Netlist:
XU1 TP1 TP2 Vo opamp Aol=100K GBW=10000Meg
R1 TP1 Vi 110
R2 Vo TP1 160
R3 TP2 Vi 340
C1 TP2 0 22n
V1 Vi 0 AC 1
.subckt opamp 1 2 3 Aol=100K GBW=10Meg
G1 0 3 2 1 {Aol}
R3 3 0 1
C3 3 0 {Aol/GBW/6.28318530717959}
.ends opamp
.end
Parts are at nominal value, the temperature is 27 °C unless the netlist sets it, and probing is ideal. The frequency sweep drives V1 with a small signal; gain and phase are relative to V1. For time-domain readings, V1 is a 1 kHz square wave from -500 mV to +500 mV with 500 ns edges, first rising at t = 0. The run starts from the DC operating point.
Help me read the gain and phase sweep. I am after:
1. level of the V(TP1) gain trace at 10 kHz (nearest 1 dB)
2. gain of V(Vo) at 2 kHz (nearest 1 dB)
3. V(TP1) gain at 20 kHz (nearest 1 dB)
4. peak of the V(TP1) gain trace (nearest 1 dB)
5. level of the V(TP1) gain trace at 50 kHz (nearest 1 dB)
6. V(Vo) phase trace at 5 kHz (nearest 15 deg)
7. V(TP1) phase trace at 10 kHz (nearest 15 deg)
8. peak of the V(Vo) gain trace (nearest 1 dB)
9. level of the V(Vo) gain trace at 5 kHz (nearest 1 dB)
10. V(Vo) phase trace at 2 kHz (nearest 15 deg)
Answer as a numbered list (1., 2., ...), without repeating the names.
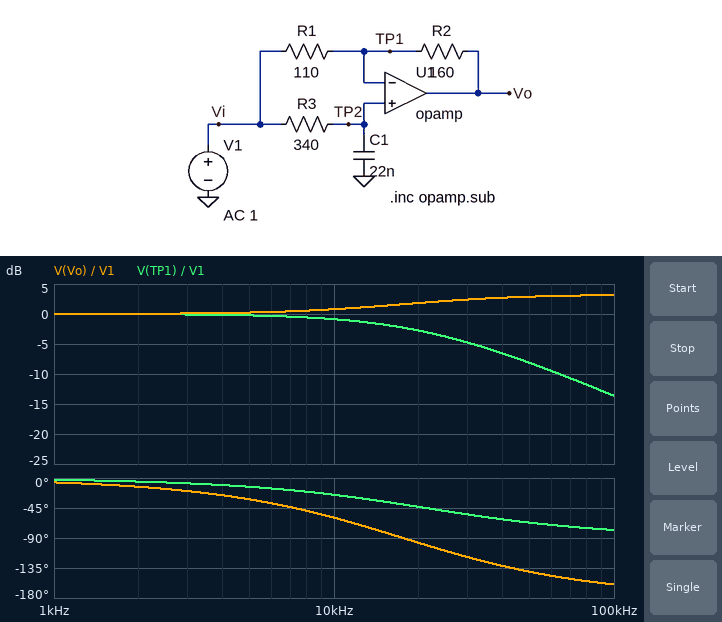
1. -1 dB
2. 0 dB
3. -3 dB
4. 0 dB
5. -8 dB
6. -30 deg
7. -30 deg
8. 3 dB
9. 0 dB
10. -15 deg
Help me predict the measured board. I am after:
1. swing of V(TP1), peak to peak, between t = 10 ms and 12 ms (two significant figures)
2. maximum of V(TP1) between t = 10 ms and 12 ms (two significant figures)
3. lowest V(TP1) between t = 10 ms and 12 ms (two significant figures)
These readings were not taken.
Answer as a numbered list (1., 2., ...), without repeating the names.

1. 1.0 V
2. 500 mV
3. -500 mV
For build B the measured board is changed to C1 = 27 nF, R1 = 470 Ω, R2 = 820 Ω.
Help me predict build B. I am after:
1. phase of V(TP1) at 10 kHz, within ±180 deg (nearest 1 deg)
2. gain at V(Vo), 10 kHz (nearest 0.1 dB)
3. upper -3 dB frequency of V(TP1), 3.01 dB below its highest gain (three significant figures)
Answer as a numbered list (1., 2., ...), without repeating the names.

1. -30 deg
2. 1.8 dB
3. 17.3 kHz
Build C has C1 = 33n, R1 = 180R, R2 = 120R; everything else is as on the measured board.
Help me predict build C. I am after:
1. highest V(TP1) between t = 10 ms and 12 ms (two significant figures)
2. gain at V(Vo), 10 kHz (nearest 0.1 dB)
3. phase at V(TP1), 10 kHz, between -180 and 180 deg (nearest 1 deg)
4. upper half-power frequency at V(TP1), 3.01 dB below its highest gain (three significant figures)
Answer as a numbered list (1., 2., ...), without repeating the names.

1. 500 mV
2. -0.9 dB
3. -35 deg
4. 14.2 kHz
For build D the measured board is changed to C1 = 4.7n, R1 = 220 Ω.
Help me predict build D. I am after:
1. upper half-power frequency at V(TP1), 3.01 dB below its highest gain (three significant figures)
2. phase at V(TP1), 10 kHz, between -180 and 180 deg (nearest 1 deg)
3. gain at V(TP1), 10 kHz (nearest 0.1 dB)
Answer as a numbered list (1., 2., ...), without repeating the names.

1. 99.6 kHz
2. -6 deg
3. 0 dB
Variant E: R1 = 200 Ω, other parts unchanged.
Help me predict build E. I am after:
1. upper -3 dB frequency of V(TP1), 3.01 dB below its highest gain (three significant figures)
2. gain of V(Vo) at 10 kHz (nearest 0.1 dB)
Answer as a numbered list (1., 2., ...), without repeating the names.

1. 21.3 kHz
2. -0.3 dB
